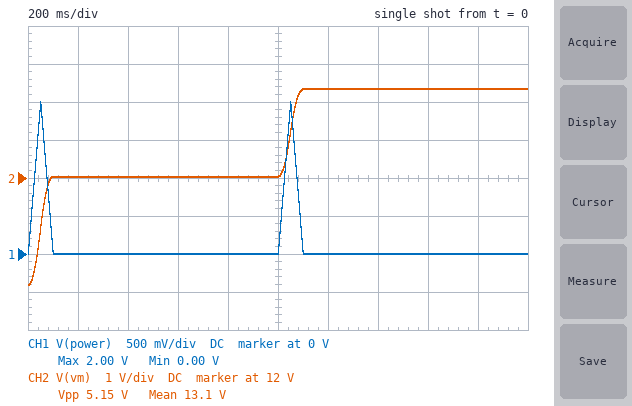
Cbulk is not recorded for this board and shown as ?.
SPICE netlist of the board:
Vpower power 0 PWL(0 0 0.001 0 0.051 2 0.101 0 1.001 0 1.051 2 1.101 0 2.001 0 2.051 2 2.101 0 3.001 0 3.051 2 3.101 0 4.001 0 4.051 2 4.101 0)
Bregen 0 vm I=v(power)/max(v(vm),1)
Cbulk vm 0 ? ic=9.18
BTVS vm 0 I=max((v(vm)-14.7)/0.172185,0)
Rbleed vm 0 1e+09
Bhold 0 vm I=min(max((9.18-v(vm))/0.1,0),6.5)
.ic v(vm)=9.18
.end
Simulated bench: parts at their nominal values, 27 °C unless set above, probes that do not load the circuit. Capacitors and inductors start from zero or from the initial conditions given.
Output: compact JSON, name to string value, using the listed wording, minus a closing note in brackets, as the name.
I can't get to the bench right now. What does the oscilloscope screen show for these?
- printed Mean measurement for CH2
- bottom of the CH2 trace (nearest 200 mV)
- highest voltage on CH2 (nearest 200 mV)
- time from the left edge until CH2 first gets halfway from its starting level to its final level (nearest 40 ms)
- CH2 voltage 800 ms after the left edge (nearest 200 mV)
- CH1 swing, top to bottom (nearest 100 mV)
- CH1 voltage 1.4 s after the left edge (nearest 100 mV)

{"printed Mean measurement for CH2": "13.1 V", "bottom of the CH2 trace": "9.2 V", "highest voltage on CH2": "14.4 V", "time from the left edge until CH2 first gets halfway from its starting level to its final level": "80 ms", "CH2 voltage 800 ms after the left edge": "12.0 V", "CH1 swing, top to bottom": "2.0 V", "CH1 voltage 1.4 s after the left edge": "0 V"}
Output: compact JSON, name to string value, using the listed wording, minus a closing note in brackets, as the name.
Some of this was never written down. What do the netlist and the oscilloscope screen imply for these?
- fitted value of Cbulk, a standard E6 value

{"fitted value of Cbulk, a standard E6 value": "3.3 mF"}
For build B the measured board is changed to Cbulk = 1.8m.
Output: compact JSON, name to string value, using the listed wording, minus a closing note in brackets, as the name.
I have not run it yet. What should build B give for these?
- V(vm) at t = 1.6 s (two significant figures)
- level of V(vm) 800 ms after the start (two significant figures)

{"V(vm) at t = 1.6 s": "15 V", "level of V(vm) 800 ms after the start": "14 V"}
